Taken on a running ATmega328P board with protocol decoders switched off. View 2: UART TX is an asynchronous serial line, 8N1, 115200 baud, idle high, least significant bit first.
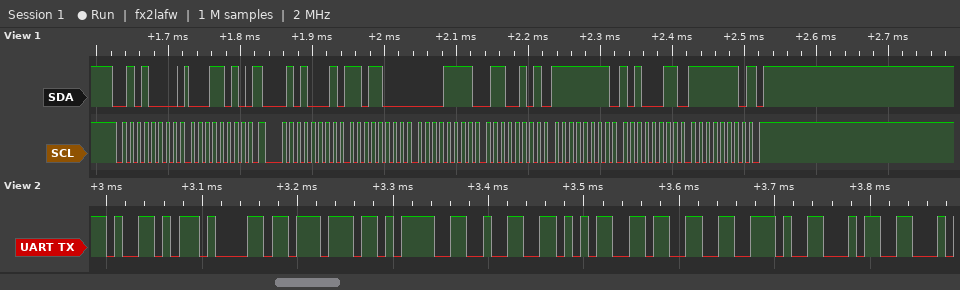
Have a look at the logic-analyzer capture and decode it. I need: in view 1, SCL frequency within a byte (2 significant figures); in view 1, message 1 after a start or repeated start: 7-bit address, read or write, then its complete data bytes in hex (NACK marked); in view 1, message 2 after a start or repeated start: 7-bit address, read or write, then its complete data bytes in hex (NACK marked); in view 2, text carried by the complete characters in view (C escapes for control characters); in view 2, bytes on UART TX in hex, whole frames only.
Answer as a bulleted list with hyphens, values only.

- 100 kHz
- 0x28 write: 1A
- 0x28 read: D8 0F 65 FF A3 FE NACK
- "Yaw=253.4"
- 59 61 77 3D 32 35 33 2E 34
